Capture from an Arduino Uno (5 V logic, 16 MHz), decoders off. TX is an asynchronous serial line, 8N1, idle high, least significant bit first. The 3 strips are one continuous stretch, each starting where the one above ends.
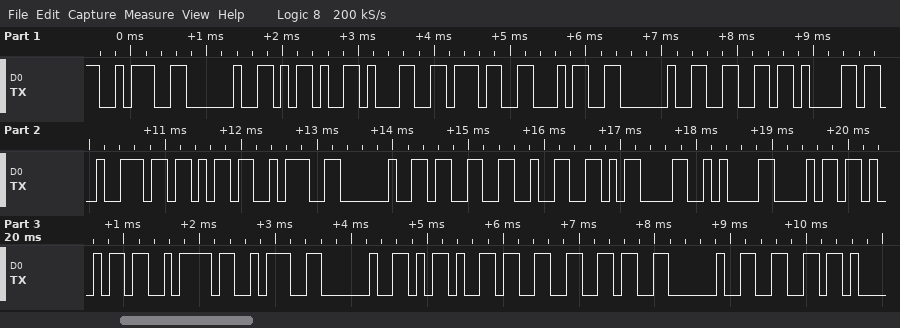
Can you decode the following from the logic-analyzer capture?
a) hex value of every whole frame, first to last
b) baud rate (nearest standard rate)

3A 20 2D 31 37 34 20 66 61 72 6B 3A 20 33 32 0D 0A 68 69 7A 3A 20 2D 33 36 20 66
9600 baud
